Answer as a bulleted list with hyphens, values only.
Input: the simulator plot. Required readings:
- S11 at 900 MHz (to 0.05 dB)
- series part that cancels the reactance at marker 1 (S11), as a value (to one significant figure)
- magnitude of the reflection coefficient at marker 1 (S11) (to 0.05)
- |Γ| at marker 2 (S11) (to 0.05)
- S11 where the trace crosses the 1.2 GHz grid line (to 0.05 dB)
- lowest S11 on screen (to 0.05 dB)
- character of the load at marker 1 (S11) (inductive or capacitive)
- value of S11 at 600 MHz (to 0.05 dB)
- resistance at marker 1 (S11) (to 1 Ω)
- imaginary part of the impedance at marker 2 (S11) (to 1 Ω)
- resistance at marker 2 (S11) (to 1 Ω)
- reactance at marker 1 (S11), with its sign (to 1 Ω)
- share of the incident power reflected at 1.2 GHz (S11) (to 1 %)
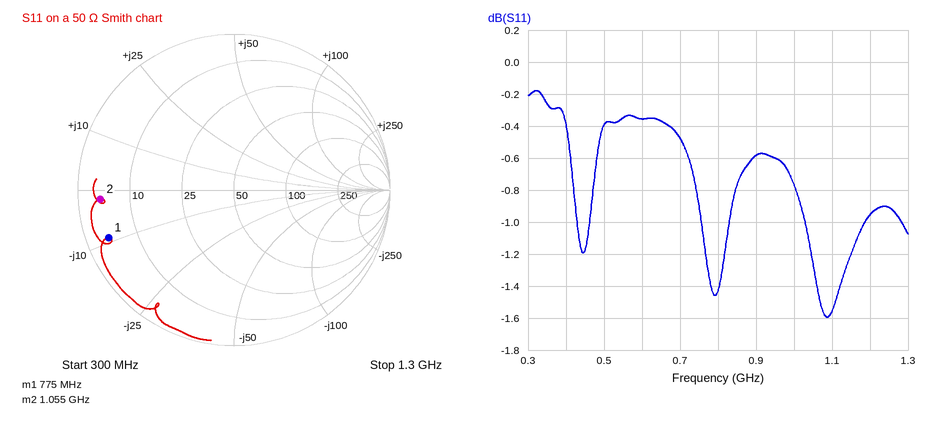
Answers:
- -0.60 dB
- 2 nH
- 0.85
- 0.85
- -0.95 dB
- -1.60 dB
- capacitive
- -0.35 dB
- 4 Ω
- -2 Ω
- 4 Ω
- -9 Ω
- 80 %
